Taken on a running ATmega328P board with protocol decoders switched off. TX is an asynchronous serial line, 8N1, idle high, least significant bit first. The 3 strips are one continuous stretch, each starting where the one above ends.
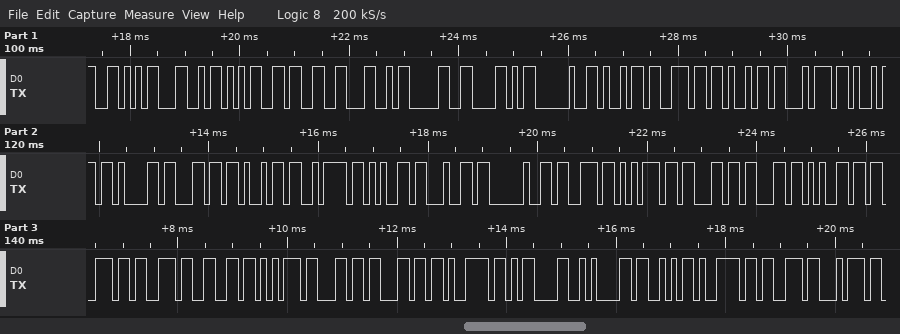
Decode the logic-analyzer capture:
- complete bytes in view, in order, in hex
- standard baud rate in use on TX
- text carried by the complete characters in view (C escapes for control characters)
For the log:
56 4C 35 33 4C 30 58 20 69 6E 69 74 69 61 6C 69 7A 65 64 20 73 75 63 63 65 73 73 66 75 6C 6C 79 0D 0A 53 79 73 74
9600 baud
"VL53L0X initialized successfully\r\nSyst"
